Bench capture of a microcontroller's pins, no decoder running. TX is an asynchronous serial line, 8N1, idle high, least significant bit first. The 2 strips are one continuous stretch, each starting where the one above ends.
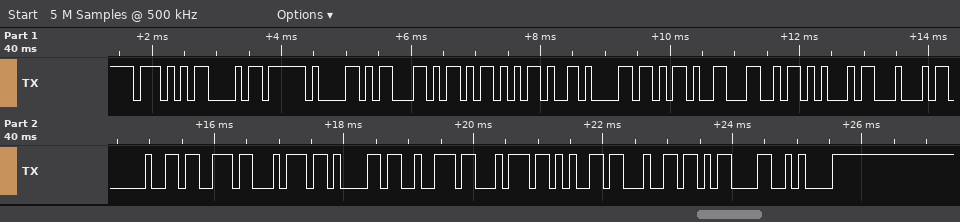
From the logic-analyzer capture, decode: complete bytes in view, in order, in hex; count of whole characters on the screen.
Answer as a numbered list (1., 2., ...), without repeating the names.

1. 0x57 0x68 0x61 0x63 0x6B 0x2D 0x61 0x2D 0x4C 0x45 0x44 0x20 0x73 0x74 0x61 0x72 0x74 0x65 0x64 0x0D 0x0A
2. 21
